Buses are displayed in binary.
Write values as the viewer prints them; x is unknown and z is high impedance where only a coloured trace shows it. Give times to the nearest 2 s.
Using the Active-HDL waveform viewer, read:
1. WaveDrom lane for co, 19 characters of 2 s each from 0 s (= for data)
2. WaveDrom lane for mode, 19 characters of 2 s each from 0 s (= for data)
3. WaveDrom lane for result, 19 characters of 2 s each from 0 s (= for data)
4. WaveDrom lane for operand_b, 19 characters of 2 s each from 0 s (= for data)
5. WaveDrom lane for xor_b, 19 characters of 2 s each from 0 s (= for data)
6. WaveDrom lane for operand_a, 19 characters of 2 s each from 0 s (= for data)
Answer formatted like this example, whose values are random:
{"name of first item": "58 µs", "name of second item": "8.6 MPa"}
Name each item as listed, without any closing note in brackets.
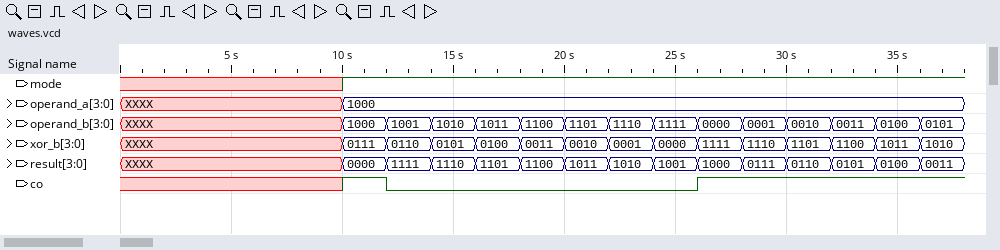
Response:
{"WaveDrom lane for co, 19 characters of 2 s each from 0 s": "{name: 'co', wave: 'x....10......1.....'}", "WaveDrom lane for mode, 19 characters of 2 s each from 0 s": "{name: 'mode', wave: 'x....1.............'}", "WaveDrom lane for result, 19 characters of 2 s each from 0 s": "{name: 'result', wave: 'x....==============', data: '0000 1111 1110 1101 1100 1011 1010 1001 1000 0111 0110 0101 0100 0011'}", "WaveDrom lane for operand_b, 19 characters of 2 s each from 0 s": "{name: 'operand_b', wave: 'x....==============', data: '1000 1001 1010 1011 1100 1101 1110 1111 0000 0001 0010 0011 0100 0101'}", "WaveDrom lane for xor_b, 19 characters of 2 s each from 0 s": "{name: 'xor_b', wave: 'x....==============', data: '0111 0110 0101 0100 0011 0010 0001 0000 1111 1110 1101 1100 1011 1010'}", "WaveDrom lane for operand_a, 19 characters of 2 s each from 0 s": "{name: 'operand_a', wave: 'x....=.............', data: '1000'}"}
